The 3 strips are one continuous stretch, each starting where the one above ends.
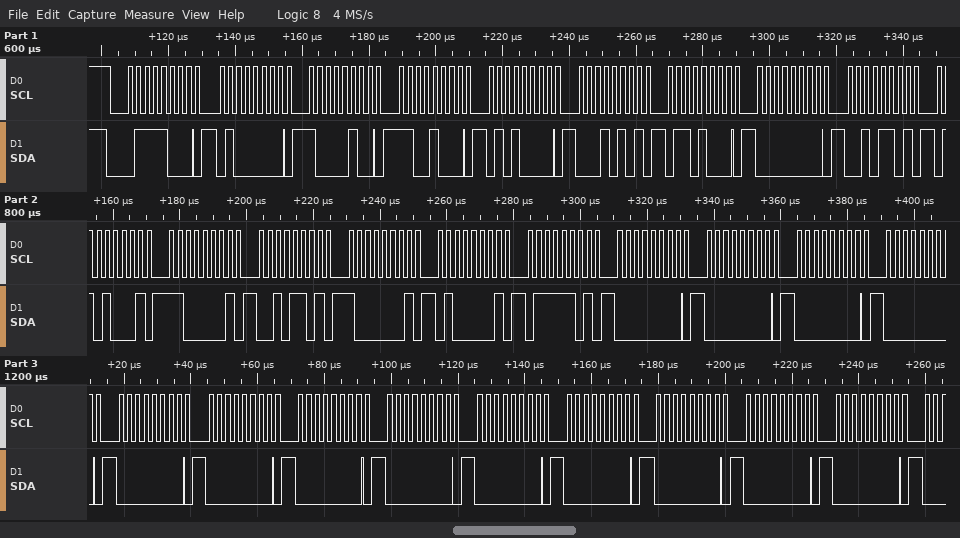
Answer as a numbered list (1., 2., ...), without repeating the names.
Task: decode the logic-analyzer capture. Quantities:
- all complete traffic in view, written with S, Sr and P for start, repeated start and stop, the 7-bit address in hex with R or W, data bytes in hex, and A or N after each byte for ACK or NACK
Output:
1. S 3CW A 40 A 84 A C8 A 50 A 15 A 68 A 00 A 2D A 51 A C1 A 2D A 81 A 41 A 7D A 00 A 00 A 00 A 00 A 00 A 00 A 00 A 00 A 00 A 00 A 00 A 00 A 00 A
